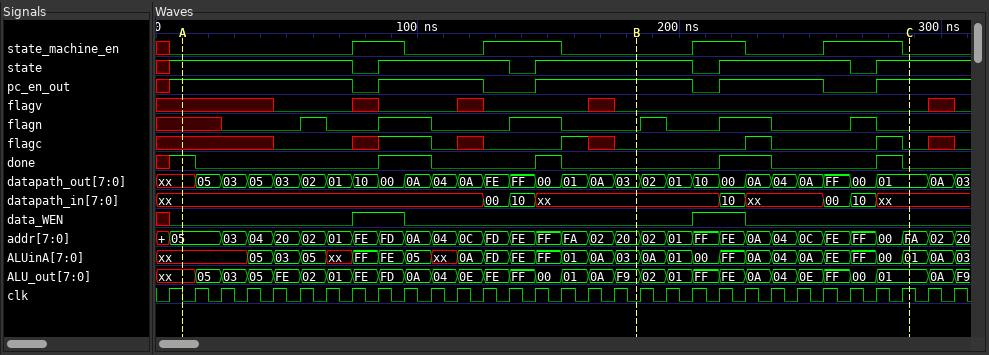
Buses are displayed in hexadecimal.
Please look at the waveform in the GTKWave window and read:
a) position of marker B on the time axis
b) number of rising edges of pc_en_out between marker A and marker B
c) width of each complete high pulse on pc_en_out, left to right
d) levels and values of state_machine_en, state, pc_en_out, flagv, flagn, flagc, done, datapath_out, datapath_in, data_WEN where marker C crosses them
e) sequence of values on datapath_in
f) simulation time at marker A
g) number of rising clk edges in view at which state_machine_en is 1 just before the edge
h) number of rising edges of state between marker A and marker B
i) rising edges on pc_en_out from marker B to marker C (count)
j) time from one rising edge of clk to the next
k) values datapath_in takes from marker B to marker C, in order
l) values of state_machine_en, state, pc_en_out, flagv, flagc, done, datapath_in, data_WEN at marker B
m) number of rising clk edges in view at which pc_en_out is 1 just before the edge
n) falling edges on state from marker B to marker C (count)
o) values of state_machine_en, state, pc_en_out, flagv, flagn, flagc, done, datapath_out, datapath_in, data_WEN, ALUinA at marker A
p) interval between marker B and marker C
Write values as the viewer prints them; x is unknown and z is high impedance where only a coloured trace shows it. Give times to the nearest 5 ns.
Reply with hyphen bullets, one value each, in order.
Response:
- 185 ns
- 2
- 40 ns, 60 ns, 40 ns
- state_machine_en=0, state=1, pc_en_out=1, flagv=0, flagn=0, flagc=0, done=0, datapath_out=01, datapath_in=xx, data_WEN=0
- xx, 00, 10, xx, 10, xx, 00, 10, xx
- 10 ns
- 10
- 2
- 2
- 10 ns
- xx, 10, xx, 00, 10, xx
- state_machine_en=0, state=1, pc_en_out=1, flagv=0, flagc=0, done=0, datapath_in=xx, data_WEN=0
- 24
- 2
- state_machine_en=0, state=1, pc_en_out=1, flagv=x, flagn=x, flagc=x, done=1, datapath_out=xx, datapath_in=xx, data_WEN=0, ALUinA=xx
- 105 ns
